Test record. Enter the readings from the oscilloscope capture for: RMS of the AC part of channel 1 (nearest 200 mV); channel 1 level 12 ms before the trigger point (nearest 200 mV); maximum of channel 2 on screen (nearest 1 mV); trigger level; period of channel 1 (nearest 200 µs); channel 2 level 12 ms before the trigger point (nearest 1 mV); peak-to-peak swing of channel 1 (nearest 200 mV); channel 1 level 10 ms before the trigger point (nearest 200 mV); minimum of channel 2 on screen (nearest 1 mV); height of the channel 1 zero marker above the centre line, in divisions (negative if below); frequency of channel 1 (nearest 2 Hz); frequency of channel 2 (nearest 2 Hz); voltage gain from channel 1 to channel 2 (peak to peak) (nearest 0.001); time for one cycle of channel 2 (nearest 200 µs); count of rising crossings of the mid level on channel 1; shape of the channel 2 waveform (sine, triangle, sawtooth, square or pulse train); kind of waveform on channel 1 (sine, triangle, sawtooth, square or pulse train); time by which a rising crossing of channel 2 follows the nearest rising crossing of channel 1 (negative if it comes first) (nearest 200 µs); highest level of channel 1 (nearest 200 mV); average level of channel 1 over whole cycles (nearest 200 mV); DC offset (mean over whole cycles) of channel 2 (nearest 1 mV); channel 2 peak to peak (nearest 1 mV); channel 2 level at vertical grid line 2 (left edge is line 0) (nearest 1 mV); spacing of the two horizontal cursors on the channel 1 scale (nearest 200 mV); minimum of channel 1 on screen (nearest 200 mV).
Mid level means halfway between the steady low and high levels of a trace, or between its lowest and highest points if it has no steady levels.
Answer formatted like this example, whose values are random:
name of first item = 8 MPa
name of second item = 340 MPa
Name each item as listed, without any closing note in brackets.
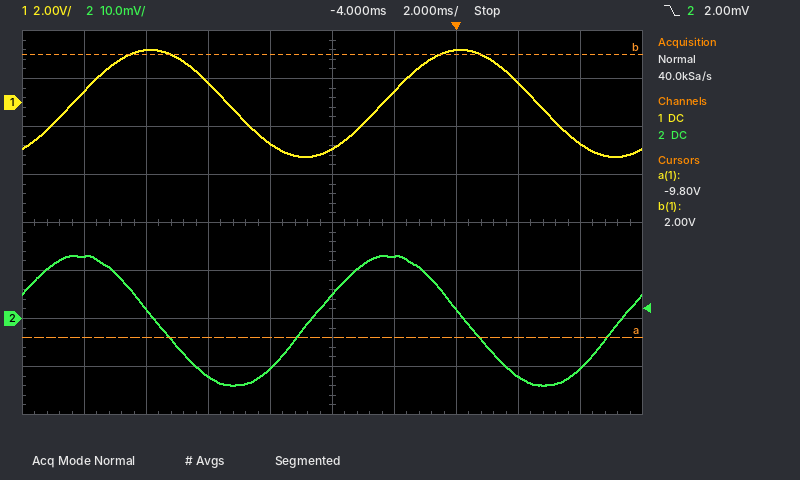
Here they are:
RMS of the AC part of channel 1 = 1.6 V
channel 1 level 12 ms before the trigger point = 400 mV
maximum of channel 2 on screen = 13 mV
trigger level = 2.00 mV
period of channel 1 = 10.0 ms
channel 2 level 12 ms before the trigger point = 13 mV
peak-to-peak swing of channel 1 = 4.4 V
channel 1 level 10 ms before the trigger point = 2.2 V
minimum of channel 2 on screen = -14 mV
height of the channel 1 zero marker above the centre line, in divisions = +2.5 div
frequency of channel 1 = 100 Hz
frequency of channel 2 = 100 Hz
voltage gain from channel 1 to channel 2 (peak to peak) = 0.006
time for one cycle of channel 2 = 10.0 ms
count of rising crossings of the mid level on channel 1 = 2
shape of the channel 2 waveform = sine
kind of waveform on channel 1 = sine
time by which a rising crossing of channel 2 follows the nearest rising crossing of channel 1 (negative if it comes first) = -2.4 ms
highest level of channel 1 = 2.2 V
average level of channel 1 over whole cycles = 0.0 V
DC offset (mean over whole cycles) of channel 2 = 0 mV
channel 2 peak to peak = 27 mV
channel 2 level at vertical grid line 2 (left edge is line 0) = 2 mV
spacing of the two horizontal cursors on the channel 1 scale = 11.8 V
minimum of channel 1 on screen = -2.2 V
